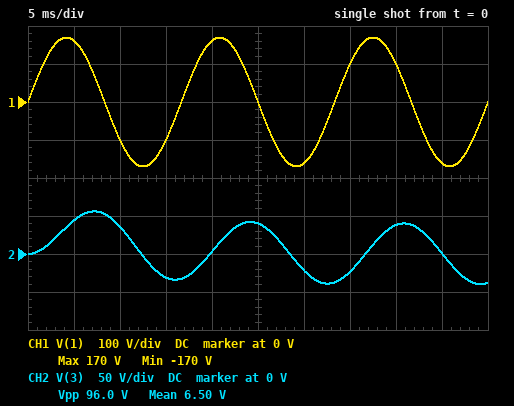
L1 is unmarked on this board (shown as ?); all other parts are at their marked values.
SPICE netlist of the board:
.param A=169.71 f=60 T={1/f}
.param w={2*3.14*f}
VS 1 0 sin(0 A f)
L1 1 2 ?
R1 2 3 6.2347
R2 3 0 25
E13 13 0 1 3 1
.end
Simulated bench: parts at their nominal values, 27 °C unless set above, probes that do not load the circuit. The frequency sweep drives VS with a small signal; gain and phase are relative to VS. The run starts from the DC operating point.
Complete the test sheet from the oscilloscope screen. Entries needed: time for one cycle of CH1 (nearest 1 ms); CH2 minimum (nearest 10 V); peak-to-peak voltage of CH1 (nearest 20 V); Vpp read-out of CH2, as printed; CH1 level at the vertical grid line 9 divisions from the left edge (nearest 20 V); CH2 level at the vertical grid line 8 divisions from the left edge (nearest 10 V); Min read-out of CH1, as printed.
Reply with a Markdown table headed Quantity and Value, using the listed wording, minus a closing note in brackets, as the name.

| Quantity | Value |
|---|---|
| time for one cycle of CH1 | 17 ms |
| CH2 minimum | -40 V |
| peak-to-peak voltage of CH1 | 340 V |
| Vpp read-out of CH2, as printed | 96.0 V |
| CH1 level at the vertical grid line 9 divisions from the left edge | -160 V |
| CH2 level at the vertical grid line 8 divisions from the left edge | 40 V |
| Min read-out of CH1, as printed | -170 V |
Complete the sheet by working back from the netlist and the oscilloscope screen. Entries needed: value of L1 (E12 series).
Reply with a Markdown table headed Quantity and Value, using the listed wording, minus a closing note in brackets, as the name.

| Quantity | Value |
|---|---|
| value of L1 | 270 mH |
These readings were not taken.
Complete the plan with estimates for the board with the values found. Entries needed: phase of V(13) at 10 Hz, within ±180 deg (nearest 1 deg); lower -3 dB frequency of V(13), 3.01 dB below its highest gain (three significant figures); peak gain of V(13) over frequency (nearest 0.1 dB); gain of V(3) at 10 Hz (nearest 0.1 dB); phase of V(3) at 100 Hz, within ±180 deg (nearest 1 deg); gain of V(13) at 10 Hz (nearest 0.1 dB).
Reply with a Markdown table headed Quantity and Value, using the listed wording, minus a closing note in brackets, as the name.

| Quantity | Value |
|---|---|
| phase of V(13) at 10 Hz, within ±180 deg | 41 deg |
| lower -3 dB frequency of V(13), 3.01 dB below its highest gain | 17.7 Hz |
| peak gain of V(13) over frequency | 0 dB |
| gain of V(3) at 10 Hz | -3.1 dB |
| phase of V(3) at 100 Hz, within ±180 deg | -80 deg |
| gain of V(13) at 10 Hz | -5.9 dB |
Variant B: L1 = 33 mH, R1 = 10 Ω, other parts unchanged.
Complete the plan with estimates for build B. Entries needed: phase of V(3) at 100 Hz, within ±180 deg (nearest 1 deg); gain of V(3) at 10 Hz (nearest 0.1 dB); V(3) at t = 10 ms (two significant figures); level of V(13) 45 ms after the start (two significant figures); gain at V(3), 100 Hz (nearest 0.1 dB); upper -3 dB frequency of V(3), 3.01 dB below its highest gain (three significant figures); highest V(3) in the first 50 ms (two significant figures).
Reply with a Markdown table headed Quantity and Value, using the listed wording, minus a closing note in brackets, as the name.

| Quantity | Value |
|---|---|
| phase of V(3) at 100 Hz, within ±180 deg | -31 deg |
| gain of V(3) at 10 Hz | -2.9 dB |
| V(3) at t = 10 ms | -32 V |
| level of V(13) 45 ms after the start | -71 V |
| gain at V(3), 100 Hz | -4.2 dB |
| upper -3 dB frequency of V(3), 3.01 dB below its highest gain | 169 Hz |
| highest V(3) in the first 50 ms | 110 V |
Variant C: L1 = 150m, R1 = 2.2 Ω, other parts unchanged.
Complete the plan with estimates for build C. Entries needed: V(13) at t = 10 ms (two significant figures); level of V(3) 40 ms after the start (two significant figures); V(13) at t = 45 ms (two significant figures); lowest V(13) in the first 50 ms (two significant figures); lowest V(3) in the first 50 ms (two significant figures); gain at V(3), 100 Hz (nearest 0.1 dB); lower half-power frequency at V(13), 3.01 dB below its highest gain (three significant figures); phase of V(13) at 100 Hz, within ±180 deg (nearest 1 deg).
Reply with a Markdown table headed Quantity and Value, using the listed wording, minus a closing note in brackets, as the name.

| Quantity | Value |
|---|---|
| V(13) at t = 10 ms | -140 V |
| level of V(3) 40 ms after the start | 67 V |
| V(13) at t = 45 ms | -150 V |
| lowest V(13) in the first 50 ms | -160 V |
| lowest V(3) in the first 50 ms | -68 V |
| gain at V(3), 100 Hz | -11.9 dB |
| lower half-power frequency at V(13), 3.01 dB below its highest gain | 28.7 Hz |
| phase of V(13) at 100 Hz, within ±180 deg | 15 deg |
